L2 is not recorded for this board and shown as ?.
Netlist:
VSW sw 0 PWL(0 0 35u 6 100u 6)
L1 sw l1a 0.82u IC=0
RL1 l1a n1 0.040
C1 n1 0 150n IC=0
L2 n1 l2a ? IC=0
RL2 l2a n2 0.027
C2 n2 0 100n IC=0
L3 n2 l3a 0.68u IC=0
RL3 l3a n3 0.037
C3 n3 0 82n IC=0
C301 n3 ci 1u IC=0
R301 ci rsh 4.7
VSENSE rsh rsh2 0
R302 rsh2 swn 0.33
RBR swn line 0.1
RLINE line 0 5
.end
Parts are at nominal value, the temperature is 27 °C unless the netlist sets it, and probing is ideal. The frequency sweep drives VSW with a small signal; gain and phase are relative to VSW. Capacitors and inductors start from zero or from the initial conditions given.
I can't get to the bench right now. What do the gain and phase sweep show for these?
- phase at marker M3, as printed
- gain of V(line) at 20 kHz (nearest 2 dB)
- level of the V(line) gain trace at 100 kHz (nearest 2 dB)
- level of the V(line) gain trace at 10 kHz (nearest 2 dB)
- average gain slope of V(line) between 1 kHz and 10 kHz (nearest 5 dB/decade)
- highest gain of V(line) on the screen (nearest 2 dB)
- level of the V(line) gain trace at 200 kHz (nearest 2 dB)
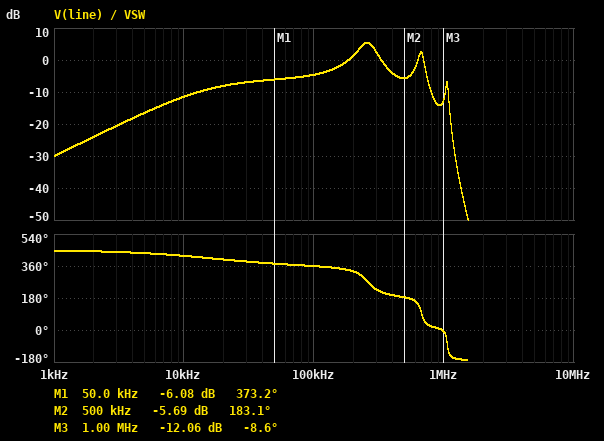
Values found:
-8.6 deg
-8 dB
-4 dB
-12 dB
20 dB/decade
6 dB
2 dB
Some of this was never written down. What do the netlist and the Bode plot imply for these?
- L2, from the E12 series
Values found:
680 nH
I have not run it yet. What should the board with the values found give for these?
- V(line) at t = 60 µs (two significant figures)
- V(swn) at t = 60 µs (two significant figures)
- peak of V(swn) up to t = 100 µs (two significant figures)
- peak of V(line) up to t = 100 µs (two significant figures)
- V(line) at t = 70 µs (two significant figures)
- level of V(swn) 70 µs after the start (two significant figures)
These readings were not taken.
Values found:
70 mV
71 mV
850 mV
830 mV
26 mV
26 mV
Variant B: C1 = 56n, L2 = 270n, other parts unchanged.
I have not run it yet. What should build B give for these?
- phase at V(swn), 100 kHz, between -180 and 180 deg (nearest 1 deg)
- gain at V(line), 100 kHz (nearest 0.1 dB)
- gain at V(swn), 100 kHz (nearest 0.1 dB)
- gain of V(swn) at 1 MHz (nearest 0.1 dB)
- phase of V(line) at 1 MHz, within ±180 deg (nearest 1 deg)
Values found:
1 deg
-5.2 dB
-5.0 dB
-12.6 dB
30 deg
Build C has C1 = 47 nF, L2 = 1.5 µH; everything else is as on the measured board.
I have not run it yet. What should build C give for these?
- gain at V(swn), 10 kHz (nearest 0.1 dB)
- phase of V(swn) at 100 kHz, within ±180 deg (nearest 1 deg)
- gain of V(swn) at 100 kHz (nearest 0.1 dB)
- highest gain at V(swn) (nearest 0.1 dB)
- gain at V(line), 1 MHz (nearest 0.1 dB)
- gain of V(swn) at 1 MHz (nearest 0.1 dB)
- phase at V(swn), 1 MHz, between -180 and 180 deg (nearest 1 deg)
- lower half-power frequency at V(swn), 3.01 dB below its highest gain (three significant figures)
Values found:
-11.3 dB
-5 deg
-4.2 dB
8.2 dB
-3.6 dB
-3.4 dB
22 deg
1.07 MHz
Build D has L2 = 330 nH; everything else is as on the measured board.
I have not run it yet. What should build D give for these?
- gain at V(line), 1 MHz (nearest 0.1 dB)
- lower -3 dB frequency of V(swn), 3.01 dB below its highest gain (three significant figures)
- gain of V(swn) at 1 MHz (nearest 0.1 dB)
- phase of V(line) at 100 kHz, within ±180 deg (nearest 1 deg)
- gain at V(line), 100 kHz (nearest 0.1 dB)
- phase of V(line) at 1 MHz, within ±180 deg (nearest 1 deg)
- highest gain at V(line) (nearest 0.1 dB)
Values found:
-18.5 dB
234 kHz
-18.3 dB
1 deg
-4.8 dB
18 deg
6.3 dB
